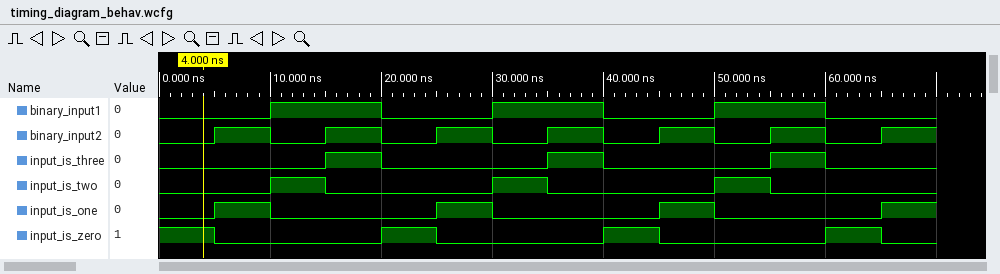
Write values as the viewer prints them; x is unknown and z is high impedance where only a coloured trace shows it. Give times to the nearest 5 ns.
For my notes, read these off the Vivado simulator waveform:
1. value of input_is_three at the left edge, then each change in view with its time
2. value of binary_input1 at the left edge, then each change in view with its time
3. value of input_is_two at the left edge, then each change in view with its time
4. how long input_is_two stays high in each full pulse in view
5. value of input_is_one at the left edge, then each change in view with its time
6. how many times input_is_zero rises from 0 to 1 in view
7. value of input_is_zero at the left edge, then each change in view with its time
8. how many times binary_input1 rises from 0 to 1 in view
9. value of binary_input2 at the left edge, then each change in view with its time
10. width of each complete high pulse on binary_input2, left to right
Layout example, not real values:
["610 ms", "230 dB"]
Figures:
["0, 1 at 15 ns, 0 at 20 ns, 1 at 35 ns, 0 at 40 ns, 1 at 55 ns, 0 at 60 ns", "0, 1 at 10 ns, 0 at 20 ns, 1 at 30 ns, 0 at 40 ns, 1 at 50 ns, 0 at 60 ns", "0, 1 at 10 ns, 0 at 15 ns, 1 at 30 ns, 0 at 35 ns, 1 at 50 ns, 0 at 55 ns", "5 ns, 5 ns, 5 ns", "0, 1 at 5 ns, 0 at 10 ns, 1 at 25 ns, 0 at 30 ns, 1 at 45 ns, 0 at 50 ns, 1 at 65 ns", "3", "1, 0 at 5 ns, 1 at 20 ns, 0 at 25 ns, 1 at 40 ns, 0 at 45 ns, 1 at 60 ns, 0 at 65 ns", "3", "0, 1 at 5 ns, 0 at 10 ns, 1 at 15 ns, 0 at 20 ns, 1 at 25 ns, 0 at 30 ns, 1 at 35 ns, 0 at 40 ns, 1 at 45 ns, 0 at 50 ns, 1 at 55 ns, 0 at 60 ns, 1 at 65 ns", "5 ns, 5 ns, 5 ns, 5 ns, 5 ns, 5 ns"]
